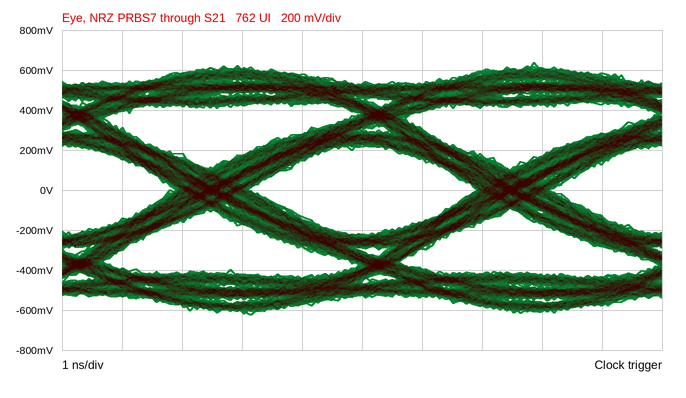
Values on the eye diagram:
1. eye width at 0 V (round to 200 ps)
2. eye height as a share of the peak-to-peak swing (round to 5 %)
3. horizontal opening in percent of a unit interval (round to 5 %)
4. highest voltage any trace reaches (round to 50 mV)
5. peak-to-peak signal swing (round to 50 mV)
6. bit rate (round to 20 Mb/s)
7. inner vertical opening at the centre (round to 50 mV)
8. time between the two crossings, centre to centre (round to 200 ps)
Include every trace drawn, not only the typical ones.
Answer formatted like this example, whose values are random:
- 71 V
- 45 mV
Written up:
- 3.8 ns
- 35 %
- 75 %
- 650 mV
- 1.25 V
- 200 Mb/s
- 450 mV
- 5.0 ns
